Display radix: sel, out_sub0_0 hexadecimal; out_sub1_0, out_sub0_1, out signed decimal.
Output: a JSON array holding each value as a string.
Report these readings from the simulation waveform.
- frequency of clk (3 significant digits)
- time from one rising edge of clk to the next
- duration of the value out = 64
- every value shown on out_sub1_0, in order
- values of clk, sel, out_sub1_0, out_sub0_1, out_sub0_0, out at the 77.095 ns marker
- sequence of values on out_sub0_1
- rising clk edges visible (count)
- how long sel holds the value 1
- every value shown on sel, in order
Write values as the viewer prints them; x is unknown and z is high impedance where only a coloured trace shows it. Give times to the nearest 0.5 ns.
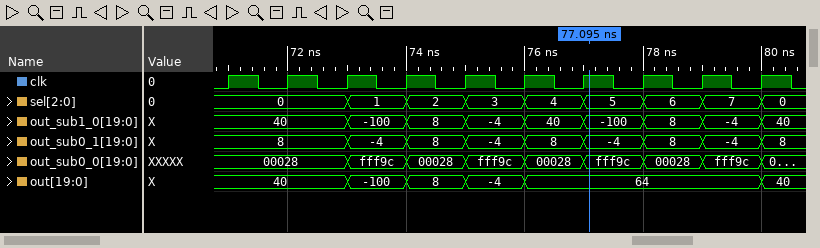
["1.00 GHz", "1 ns", "4 ns", "40, -100, 8, -4, 40, -100, 8, -4, 40", "clk=1, sel=5, out_sub1_0=-100, out_sub0_1=-4, out_sub0_0=fff9c, out=64", "8, -4, 8, -4, 8, -4, 8, -4, 8", "10", "1 ns", "0, 1, 2, 3, 4, 5, 6, 7, 0"]
